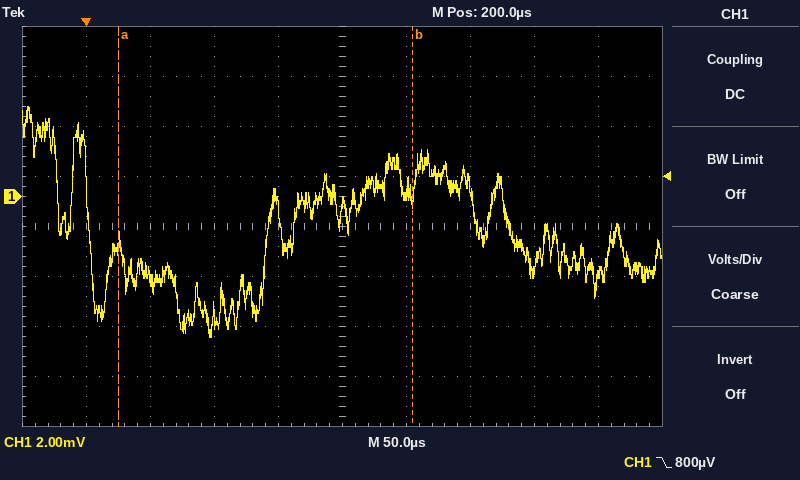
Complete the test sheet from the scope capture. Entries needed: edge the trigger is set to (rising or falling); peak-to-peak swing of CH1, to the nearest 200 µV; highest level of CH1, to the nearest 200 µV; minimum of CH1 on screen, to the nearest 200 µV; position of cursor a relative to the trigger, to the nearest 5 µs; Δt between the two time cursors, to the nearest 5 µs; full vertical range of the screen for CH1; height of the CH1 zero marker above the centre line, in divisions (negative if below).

falling
9.2 mV
3.6 mV
-5.6 mV
+25 µs
230 µs
16 mV
+0.6 div
